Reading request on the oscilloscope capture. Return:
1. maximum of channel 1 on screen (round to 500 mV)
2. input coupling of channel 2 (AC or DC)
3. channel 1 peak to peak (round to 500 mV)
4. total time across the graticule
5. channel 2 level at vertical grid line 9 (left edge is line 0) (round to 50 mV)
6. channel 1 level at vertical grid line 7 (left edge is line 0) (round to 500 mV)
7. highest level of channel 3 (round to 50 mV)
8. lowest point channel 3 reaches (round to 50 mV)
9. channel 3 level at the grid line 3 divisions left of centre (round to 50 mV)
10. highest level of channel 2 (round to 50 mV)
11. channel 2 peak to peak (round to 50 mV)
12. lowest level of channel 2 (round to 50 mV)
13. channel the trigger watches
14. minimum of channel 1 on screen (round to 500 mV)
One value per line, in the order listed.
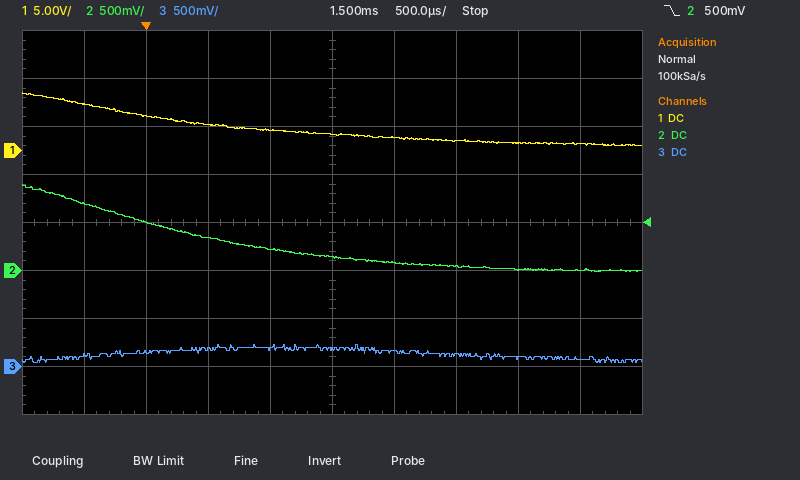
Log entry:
6.0 V
DC
5.5 V
5 ms
0 mV
1.0 V
250 mV
50 mV
150 mV
900 mV
900 mV
0 mV
channel 2
500 mV
